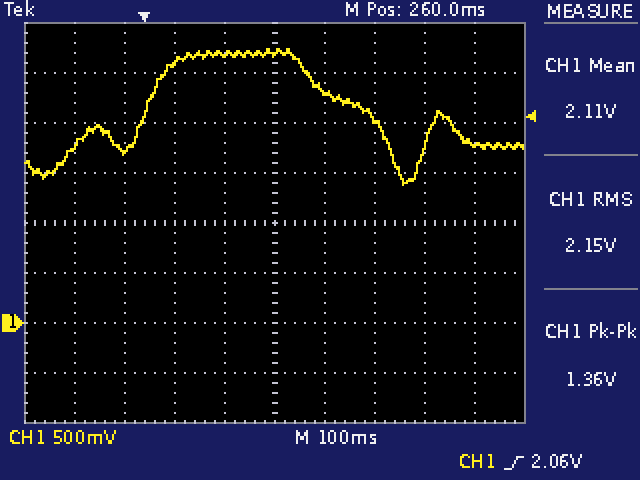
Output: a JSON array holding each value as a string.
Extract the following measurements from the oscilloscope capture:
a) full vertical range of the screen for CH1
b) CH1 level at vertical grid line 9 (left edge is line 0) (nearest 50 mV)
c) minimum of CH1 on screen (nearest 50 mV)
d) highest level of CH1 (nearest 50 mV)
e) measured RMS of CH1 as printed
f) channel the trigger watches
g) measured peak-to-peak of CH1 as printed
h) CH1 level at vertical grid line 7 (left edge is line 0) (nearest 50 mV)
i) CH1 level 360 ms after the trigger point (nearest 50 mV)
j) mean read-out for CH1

["4 V", "1.80 V", "1.40 V", "2.75 V", "2.15 V", "CH1", "1.36 V", "2.05 V", "2.30 V", "2.11 V"]
